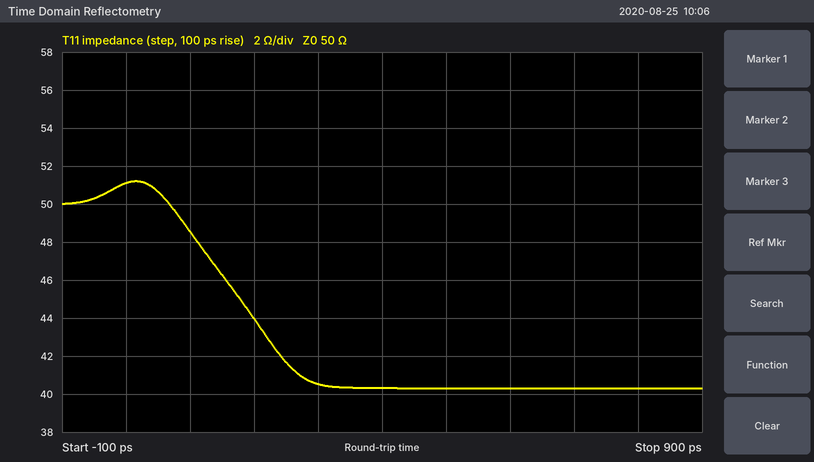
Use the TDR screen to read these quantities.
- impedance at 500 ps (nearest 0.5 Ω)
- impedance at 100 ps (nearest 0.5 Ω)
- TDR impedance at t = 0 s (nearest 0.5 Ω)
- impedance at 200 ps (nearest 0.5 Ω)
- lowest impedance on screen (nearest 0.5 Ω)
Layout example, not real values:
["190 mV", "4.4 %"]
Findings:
["40.5 Ω", "48.5 Ω", "51.0 Ω", "44.0 Ω", "40.5 Ω"]
